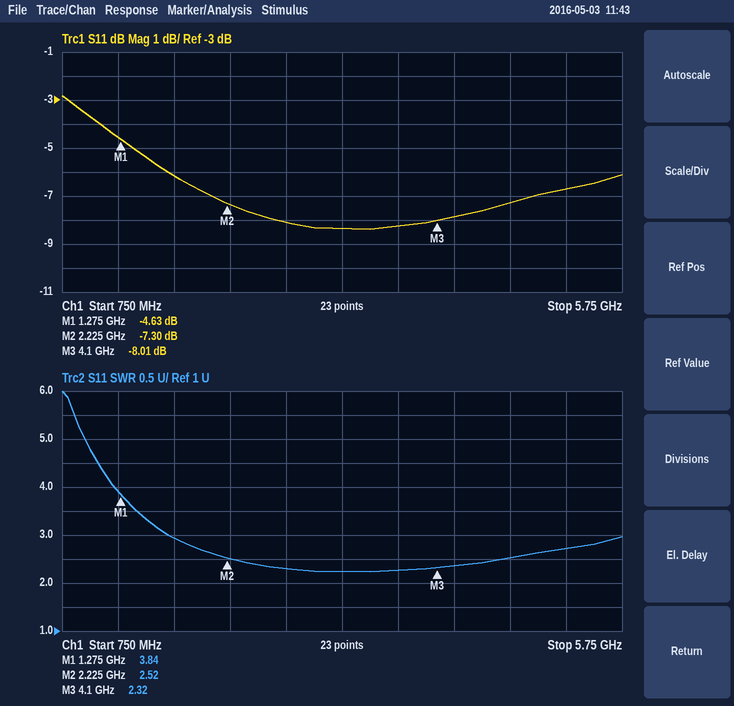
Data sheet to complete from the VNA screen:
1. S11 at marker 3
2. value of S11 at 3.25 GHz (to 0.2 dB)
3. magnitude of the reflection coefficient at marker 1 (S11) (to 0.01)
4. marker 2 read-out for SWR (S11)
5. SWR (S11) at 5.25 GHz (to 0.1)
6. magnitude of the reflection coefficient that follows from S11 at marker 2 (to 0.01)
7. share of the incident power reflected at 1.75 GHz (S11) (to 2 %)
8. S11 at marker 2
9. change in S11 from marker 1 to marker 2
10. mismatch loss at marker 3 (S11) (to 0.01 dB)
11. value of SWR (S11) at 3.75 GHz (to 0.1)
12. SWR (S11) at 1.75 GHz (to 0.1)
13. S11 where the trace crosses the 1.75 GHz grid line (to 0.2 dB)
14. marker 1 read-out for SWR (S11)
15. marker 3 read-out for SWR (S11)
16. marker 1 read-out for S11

-8.01 dB
-8.4 dB
0.59
2.52
2.7
0.43
24 %
-7.30 dB
-2.67 dB
0.75 dB
2.3
2.9
-6.2 dB
3.84
2.32
-4.63 dB
